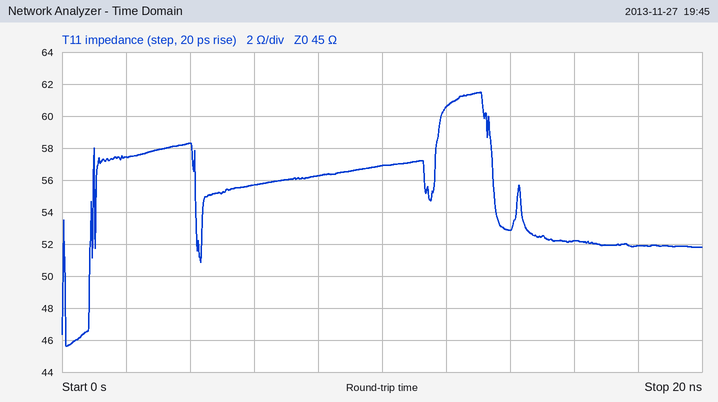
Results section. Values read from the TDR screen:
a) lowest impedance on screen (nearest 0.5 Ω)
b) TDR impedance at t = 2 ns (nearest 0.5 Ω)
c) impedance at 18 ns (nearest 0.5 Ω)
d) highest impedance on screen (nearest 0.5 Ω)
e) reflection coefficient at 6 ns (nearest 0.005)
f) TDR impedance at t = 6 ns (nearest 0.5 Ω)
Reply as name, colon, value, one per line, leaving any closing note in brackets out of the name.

lowest impedance on screen: 45.5 Ω
TDR impedance at t = 2 ns: 57.5 Ω
impedance at 18 ns: 52.0 Ω
highest impedance on screen: 61.5 Ω
reflection coefficient at 6 ns: +0.105
TDR impedance at t = 6 ns: 55.5 Ω
